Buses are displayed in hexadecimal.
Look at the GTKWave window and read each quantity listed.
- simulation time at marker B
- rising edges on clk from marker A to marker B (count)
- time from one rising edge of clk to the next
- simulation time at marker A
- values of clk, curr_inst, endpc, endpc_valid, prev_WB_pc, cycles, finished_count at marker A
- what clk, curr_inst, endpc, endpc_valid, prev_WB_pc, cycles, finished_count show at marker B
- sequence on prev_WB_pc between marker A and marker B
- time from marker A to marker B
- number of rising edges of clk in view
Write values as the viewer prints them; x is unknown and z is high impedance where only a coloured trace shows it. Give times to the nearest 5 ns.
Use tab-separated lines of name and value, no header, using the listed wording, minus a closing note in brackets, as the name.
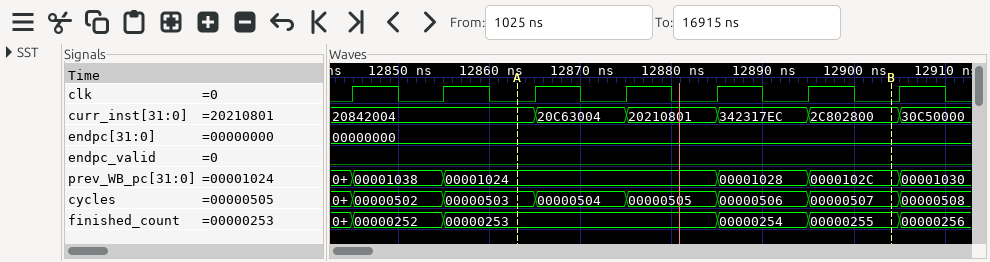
simulation time at marker B	12905 ns
rising edges on clk from marker A to marker B	4
time from one rising edge of clk to the next	10 ns
simulation time at marker A	12865 ns
values of clk, curr_inst, endpc, endpc_valid, prev_WB_pc, cycles, finished_count at marker A	clk=0, curr_inst=20842004, endpc=00000000, endpc_valid=0, prev_WB_pc=00001024, cycles=00000503, finished_count=00000253
what clk, curr_inst, endpc, endpc_valid, prev_WB_pc, cycles, finished_count show at marker B	clk=0, curr_inst=2C802800, endpc=00000000, endpc_valid=0, prev_WB_pc=0000102C, cycles=00000507, finished_count=00000255
sequence on prev_WB_pc between marker A and marker B	00001024, 00001028, 0000102C
time from marker A to marker B	40 ns
number of rising edges of clk in view	7
